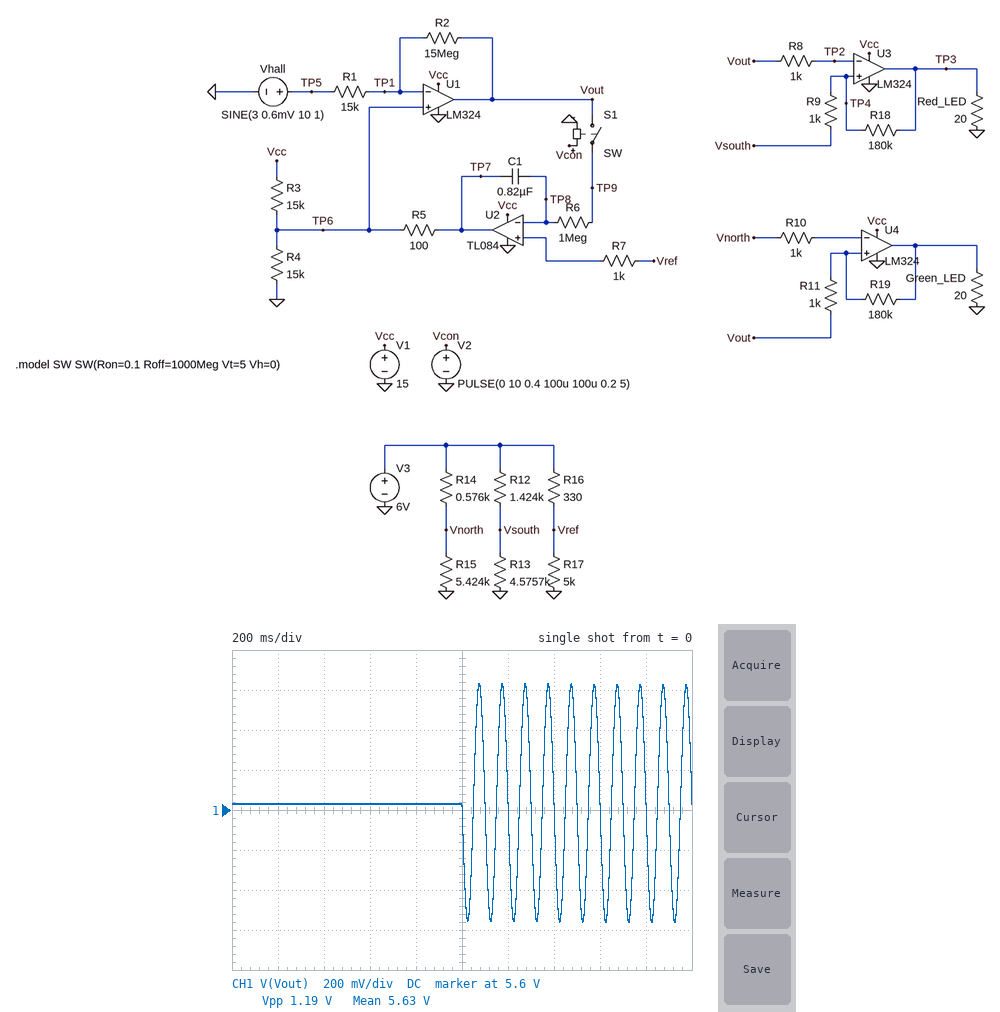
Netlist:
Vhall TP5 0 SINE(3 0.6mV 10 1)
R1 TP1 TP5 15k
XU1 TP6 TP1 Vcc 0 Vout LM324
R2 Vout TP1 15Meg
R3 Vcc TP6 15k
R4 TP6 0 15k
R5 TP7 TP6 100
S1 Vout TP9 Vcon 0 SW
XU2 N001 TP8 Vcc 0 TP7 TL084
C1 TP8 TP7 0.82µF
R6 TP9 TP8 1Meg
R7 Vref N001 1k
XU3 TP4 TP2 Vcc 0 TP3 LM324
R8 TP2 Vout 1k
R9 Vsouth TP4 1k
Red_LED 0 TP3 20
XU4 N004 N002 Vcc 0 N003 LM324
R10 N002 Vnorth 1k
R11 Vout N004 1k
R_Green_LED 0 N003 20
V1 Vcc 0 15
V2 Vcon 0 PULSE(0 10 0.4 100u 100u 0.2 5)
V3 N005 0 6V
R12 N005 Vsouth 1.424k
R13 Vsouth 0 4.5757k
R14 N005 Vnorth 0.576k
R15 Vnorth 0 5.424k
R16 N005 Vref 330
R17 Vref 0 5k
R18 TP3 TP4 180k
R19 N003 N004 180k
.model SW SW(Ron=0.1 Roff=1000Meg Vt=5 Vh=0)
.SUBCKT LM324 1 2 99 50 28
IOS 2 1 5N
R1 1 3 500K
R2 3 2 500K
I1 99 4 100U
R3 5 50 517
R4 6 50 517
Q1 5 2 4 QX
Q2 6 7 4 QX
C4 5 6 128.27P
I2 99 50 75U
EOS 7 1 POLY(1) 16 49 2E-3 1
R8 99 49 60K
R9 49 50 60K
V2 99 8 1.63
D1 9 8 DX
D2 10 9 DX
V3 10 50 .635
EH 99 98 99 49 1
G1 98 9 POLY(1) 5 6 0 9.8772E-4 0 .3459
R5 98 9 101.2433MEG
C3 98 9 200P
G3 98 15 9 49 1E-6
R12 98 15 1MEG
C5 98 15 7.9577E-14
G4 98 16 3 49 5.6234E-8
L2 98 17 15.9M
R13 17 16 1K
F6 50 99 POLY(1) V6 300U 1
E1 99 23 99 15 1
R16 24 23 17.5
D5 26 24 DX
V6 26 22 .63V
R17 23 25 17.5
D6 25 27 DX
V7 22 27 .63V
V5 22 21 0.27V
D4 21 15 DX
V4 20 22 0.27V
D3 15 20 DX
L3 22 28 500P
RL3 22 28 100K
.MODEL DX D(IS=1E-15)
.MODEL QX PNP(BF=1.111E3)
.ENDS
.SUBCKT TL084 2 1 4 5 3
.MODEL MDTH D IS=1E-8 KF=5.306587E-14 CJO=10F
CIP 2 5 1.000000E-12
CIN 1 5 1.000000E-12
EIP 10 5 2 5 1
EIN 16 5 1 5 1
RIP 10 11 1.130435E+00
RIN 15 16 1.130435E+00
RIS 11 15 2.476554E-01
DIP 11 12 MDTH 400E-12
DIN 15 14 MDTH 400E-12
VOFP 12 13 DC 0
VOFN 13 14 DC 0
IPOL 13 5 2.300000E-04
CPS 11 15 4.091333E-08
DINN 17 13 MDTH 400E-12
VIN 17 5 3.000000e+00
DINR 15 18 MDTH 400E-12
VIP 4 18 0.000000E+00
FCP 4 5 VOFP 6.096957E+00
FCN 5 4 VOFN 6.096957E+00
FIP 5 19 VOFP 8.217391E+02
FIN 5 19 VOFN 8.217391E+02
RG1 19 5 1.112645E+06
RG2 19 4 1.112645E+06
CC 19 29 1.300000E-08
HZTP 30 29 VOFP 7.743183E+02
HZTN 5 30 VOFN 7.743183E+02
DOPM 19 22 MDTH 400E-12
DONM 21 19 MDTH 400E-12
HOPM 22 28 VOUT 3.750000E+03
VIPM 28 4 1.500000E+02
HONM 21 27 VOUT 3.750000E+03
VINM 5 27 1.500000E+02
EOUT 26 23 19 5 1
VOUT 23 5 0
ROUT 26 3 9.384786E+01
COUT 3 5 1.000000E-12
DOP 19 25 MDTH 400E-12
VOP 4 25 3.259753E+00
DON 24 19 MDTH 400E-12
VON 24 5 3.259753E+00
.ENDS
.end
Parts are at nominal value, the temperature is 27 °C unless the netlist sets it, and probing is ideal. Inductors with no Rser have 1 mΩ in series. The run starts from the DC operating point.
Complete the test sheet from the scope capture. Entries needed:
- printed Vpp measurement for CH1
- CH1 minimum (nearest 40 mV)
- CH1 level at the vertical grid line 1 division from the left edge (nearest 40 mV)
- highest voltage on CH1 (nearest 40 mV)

1.19 V
5.04 V
5.64 V
6.24 V
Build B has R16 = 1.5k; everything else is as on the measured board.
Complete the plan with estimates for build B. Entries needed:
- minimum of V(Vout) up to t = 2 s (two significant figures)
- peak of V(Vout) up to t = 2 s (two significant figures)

4.0 V
5.2 V
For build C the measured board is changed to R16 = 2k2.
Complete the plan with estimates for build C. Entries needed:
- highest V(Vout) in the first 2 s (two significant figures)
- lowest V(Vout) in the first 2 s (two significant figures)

4.8 V
3.6 V
